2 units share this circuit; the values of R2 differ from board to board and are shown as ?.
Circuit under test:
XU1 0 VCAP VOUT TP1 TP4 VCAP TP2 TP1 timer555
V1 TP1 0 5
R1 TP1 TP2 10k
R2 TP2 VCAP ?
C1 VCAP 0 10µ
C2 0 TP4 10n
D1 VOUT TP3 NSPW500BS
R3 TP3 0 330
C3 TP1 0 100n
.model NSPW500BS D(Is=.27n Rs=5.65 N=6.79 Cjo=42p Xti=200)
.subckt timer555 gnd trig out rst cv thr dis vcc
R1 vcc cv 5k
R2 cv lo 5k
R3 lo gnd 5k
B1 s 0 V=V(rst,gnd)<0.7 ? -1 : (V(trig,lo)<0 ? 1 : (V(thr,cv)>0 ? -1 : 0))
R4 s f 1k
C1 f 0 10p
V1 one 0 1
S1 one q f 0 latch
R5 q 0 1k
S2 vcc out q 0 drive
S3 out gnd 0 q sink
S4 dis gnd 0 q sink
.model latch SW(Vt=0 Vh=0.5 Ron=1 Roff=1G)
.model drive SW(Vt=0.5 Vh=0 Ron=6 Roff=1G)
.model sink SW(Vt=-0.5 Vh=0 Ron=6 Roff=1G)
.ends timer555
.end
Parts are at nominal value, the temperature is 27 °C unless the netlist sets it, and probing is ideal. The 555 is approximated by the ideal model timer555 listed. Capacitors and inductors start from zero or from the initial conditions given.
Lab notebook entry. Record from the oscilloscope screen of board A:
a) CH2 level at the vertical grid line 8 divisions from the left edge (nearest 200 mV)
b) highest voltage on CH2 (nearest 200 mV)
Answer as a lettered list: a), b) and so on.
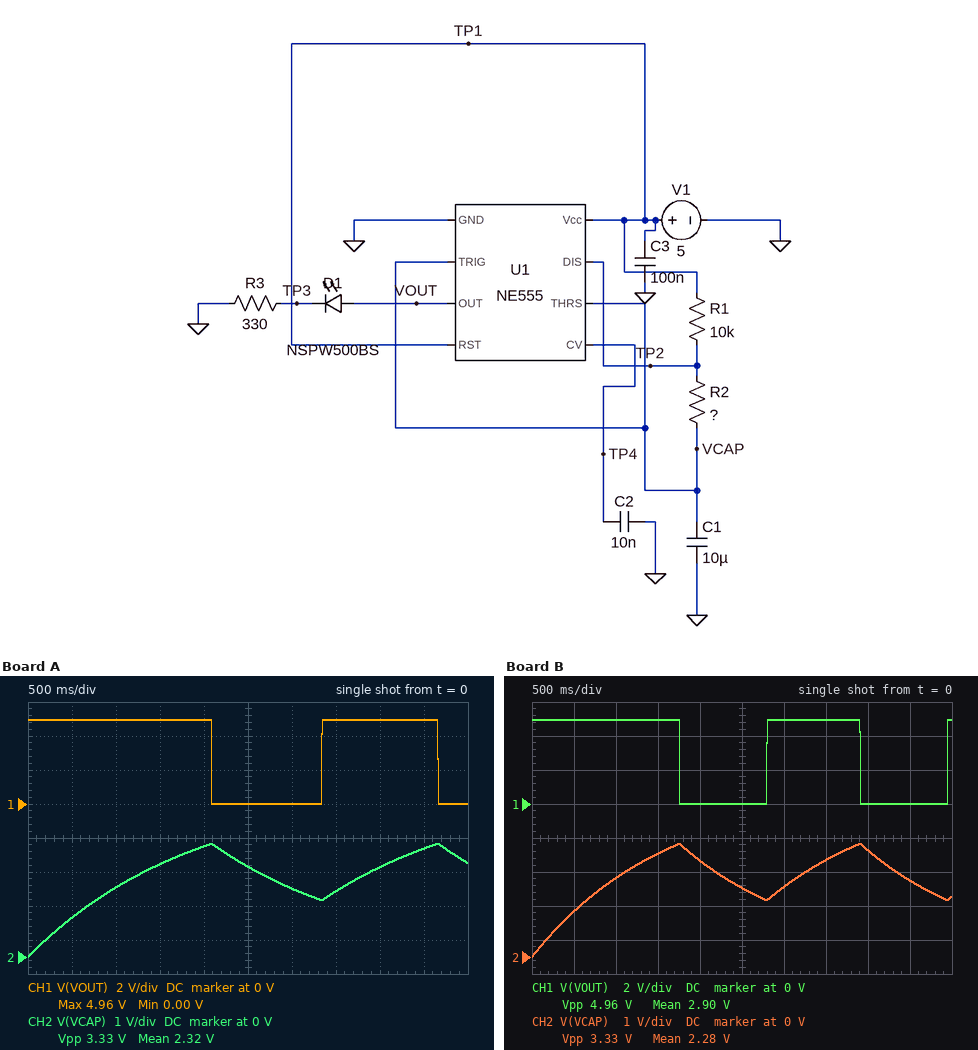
a) 2.6 V
b) 3.4 V
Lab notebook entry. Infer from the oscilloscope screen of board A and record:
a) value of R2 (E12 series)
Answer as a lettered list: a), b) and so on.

a) 180 kΩ
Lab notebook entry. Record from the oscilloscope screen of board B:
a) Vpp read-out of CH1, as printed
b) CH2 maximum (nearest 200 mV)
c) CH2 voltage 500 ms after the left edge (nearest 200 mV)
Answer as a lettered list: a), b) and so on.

a) 4.96 V
b) 3.4 V
c) 1.4 V
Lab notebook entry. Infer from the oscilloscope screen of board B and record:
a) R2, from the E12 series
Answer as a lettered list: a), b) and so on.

a) 150 kΩ
